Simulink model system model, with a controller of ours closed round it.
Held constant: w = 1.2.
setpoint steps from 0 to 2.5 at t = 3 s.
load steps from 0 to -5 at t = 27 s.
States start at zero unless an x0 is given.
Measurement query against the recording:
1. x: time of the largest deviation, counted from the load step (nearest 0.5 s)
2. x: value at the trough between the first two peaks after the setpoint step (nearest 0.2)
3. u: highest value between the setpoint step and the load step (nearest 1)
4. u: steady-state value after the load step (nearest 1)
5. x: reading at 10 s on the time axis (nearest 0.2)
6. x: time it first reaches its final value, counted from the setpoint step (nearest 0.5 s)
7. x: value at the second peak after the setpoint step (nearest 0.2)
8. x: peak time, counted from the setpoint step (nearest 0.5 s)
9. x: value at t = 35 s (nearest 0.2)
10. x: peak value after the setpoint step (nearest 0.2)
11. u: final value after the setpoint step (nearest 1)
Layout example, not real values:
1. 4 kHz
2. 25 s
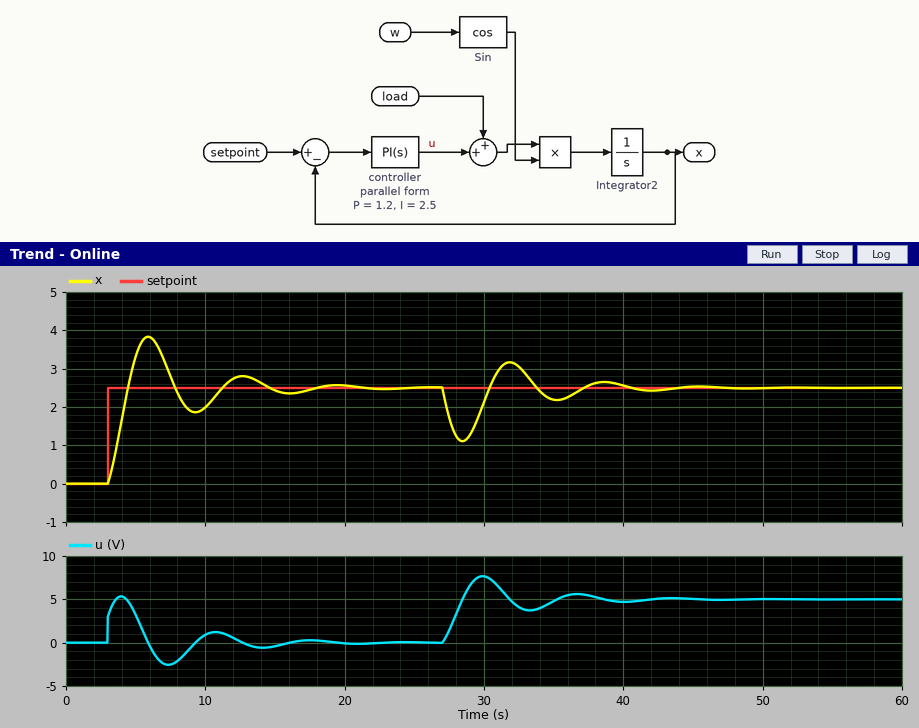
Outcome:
1. 1.5 s
2. 1.8
3. 5
4. 5
5. 2.0
6. 1.5 s
7. 2.8
8. 3.0 s
9. 2.2
10. 3.8
11. 0
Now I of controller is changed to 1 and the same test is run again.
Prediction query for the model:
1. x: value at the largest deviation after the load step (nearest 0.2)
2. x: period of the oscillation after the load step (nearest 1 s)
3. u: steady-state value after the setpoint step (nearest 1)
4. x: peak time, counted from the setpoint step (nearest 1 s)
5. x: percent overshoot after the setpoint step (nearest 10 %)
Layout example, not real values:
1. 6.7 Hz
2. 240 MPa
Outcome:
1. 0.6
2. 11 s
3. 0
4. 4 s
5. 40 %
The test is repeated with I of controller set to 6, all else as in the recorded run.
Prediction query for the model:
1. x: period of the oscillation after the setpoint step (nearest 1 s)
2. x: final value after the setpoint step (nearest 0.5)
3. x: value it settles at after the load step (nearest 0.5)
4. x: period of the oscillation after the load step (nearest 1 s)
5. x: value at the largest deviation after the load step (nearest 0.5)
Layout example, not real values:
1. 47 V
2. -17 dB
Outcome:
1. 4 s
2. 2.5
3. 2.5
4. 4 s
5. 1.5
